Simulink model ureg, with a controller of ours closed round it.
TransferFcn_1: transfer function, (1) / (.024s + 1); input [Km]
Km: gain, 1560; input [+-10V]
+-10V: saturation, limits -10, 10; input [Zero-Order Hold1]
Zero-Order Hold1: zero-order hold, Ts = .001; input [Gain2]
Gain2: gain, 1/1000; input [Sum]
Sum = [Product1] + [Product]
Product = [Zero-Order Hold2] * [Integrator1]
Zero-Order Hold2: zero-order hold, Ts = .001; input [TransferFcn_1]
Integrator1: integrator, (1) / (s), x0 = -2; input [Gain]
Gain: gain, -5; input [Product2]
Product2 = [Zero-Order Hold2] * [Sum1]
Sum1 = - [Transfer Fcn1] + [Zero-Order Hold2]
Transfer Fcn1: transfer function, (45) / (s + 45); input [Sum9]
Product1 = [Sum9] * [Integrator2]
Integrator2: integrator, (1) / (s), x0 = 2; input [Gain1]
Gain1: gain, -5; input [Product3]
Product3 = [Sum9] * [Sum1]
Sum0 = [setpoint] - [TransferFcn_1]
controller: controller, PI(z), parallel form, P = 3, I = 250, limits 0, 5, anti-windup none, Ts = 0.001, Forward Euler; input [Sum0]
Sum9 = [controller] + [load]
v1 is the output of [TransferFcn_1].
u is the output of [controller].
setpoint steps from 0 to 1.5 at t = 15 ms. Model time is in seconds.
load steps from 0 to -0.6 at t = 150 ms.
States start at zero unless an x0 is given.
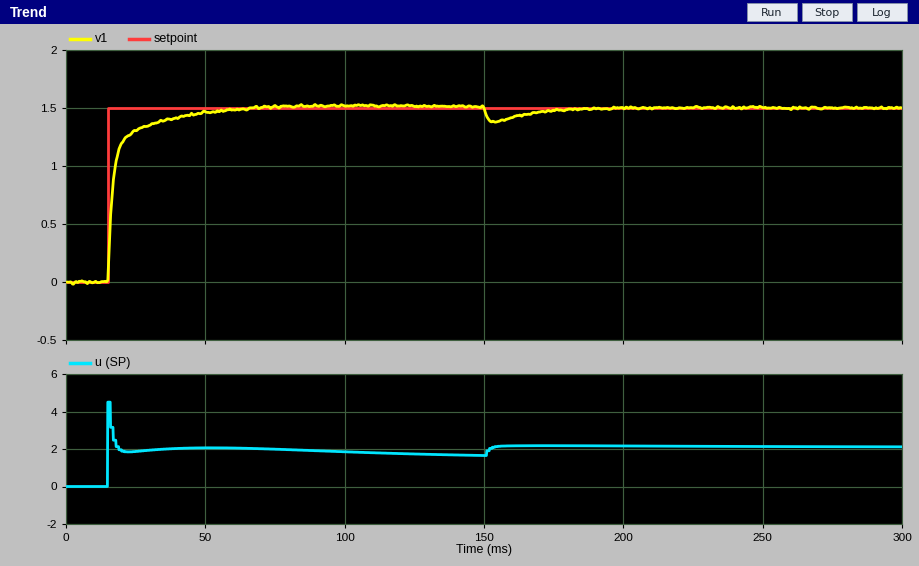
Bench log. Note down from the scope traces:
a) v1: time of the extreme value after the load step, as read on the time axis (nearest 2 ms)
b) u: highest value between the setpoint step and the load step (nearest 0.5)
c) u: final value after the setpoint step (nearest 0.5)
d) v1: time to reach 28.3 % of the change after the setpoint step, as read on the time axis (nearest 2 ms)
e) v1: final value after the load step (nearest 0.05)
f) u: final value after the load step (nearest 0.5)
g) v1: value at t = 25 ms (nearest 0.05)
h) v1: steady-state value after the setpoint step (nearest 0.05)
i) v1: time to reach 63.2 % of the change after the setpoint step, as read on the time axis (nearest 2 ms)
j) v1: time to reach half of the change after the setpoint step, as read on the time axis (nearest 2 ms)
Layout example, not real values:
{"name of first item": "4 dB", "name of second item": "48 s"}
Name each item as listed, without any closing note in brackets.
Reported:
{"v1: time of the extreme value after the load step, as read on the time axis": "154 ms", "u: highest value between the setpoint step and the load step": "4.5", "u: final value after the setpoint step": "1.5", "v1: time to reach 28.3 % of the change after the setpoint step, as read on the time axis": "16 ms", "v1: final value after the load step": "1.50", "u: final value after the load step": "2.0", "v1: value at t = 25 ms": "1.30", "v1: steady-state value after the setpoint step": "1.50", "v1: time to reach 63.2 % of the change after the setpoint step, as read on the time axis": "18 ms", "v1: time to reach half of the change after the setpoint step, as read on the time axis": "16 ms"}
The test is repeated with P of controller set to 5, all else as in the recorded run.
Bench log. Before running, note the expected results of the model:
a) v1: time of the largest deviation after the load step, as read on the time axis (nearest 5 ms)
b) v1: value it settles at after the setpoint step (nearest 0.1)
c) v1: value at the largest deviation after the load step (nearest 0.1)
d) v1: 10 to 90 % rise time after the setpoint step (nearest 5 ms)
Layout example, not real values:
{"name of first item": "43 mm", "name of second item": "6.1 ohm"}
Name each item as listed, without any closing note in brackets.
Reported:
{"v1: time of the largest deviation after the load step, as read on the time axis": "150 ms", "v1: value it settles at after the setpoint step": "1.5", "v1: value at the largest deviation after the load step": "1.4", "v1: 10 to 90 % rise time after the setpoint step": "15 ms"}
